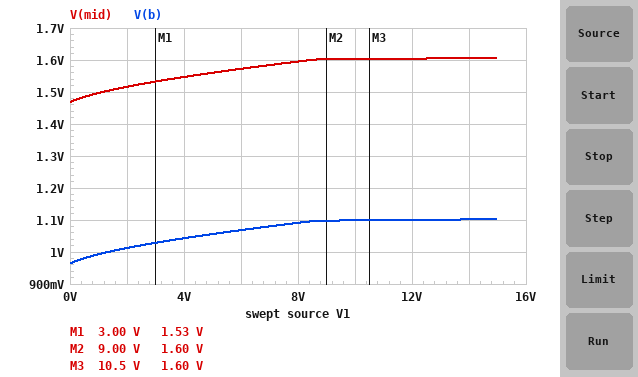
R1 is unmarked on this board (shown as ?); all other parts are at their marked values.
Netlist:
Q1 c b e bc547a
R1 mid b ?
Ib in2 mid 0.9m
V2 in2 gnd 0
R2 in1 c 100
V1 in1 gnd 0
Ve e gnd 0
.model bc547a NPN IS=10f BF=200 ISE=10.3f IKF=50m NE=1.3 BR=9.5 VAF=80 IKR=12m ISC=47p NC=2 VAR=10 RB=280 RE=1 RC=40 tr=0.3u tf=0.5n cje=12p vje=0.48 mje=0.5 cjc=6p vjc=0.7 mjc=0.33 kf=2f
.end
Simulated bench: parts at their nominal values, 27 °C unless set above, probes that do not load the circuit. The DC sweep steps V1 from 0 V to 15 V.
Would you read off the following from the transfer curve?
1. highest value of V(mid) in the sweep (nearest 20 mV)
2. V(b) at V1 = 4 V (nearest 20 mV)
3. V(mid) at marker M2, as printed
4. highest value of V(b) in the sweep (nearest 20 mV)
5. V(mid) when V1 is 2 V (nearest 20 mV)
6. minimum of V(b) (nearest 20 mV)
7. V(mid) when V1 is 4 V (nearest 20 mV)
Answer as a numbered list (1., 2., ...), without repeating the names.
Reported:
1. 1.60 V
2. 1.04 V
3. 1.60 V
4. 1.10 V
5. 1.52 V
6. 960 mV
7. 1.54 V
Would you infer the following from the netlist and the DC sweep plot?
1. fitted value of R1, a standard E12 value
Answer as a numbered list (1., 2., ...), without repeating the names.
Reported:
1. 560 Ω
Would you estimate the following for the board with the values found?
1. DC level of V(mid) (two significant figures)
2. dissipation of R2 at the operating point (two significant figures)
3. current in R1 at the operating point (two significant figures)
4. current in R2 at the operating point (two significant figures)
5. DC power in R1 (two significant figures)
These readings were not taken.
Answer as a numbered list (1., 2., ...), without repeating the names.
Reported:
1. 1.5 V
2. 130 nW
3. 900 µA
4. 36 µA
5. 450 µW
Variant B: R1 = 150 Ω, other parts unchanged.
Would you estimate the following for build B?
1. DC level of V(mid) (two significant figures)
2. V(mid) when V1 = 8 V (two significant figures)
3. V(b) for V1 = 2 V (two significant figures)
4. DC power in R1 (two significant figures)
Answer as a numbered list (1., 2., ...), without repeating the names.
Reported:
1. 1.1 V
2. 1.2 V
3. 1.0 V
4. 120 µW
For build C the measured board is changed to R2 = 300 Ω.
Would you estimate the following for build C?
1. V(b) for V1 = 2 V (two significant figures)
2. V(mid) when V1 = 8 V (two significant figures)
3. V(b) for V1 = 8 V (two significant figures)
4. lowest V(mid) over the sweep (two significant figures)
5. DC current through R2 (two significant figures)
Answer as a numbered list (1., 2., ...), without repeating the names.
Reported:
1. 990 mV
2. 1.5 V
3. 1.0 V
4. 1.5 V
5. 15 µA
